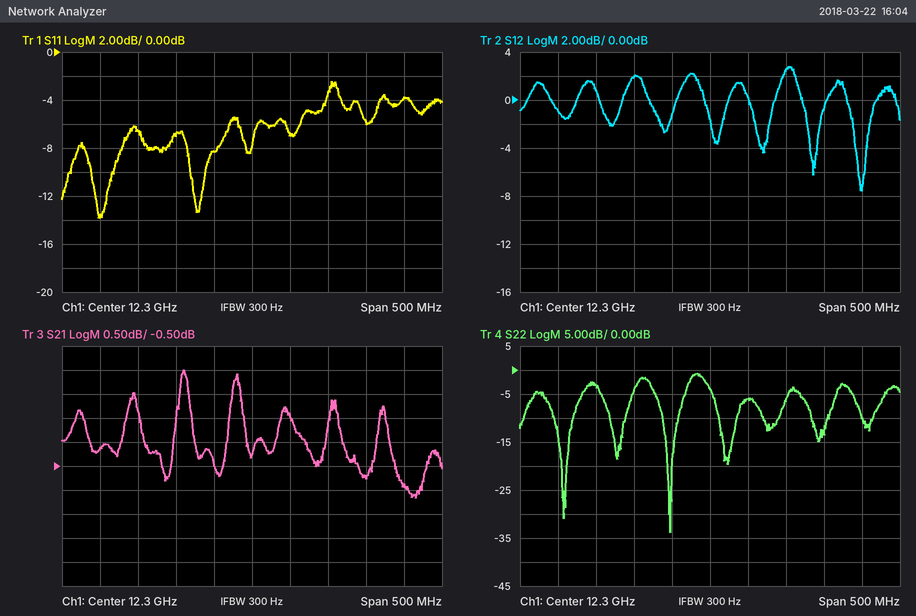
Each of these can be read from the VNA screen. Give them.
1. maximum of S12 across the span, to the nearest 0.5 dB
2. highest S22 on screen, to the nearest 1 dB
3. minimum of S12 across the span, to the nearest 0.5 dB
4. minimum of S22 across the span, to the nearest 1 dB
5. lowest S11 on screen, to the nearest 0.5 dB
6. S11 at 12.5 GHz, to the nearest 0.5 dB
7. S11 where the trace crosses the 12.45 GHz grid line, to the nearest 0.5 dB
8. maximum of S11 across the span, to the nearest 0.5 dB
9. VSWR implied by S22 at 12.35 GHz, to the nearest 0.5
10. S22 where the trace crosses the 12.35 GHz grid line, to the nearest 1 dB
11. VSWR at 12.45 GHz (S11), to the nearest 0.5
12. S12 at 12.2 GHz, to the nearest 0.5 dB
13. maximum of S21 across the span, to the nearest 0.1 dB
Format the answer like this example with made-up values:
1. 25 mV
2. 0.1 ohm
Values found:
1. 3.0 dB
2. -1 dB
3. -7.5 dB
4. -34 dB
5. -14.0 dB
6. -4.0 dB
7. -6.0 dB
8. -2.5 dB
9. 3.0
10. -6 dB
11. 3.0
12. 2.0 dB
13. 1.5 dB
